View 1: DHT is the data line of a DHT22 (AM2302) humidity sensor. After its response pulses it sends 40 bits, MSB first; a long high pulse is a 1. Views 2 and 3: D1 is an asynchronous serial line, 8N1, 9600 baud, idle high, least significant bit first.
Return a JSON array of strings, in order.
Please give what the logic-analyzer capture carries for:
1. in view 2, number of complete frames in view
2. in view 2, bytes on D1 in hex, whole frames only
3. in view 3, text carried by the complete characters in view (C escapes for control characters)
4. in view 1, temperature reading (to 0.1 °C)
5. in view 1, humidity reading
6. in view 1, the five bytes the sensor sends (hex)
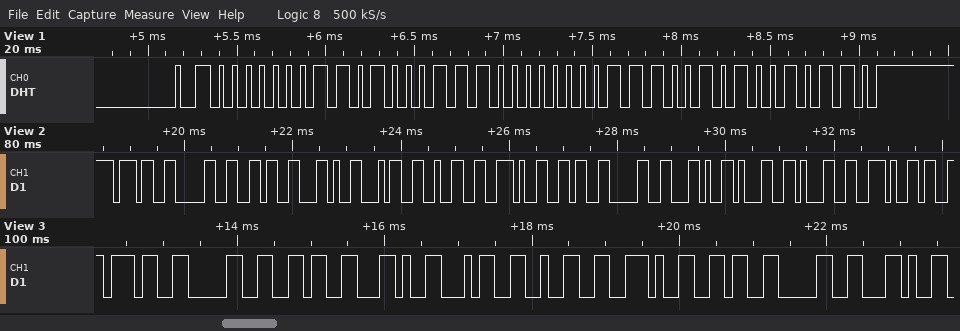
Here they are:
["13", "37 30 36 2C 34 32 2E 36 30 2C 31 31 2E", "\"706,42.60,\"", "-11.4 °C", "41.9 %", "01 A3 80 72 96"]
